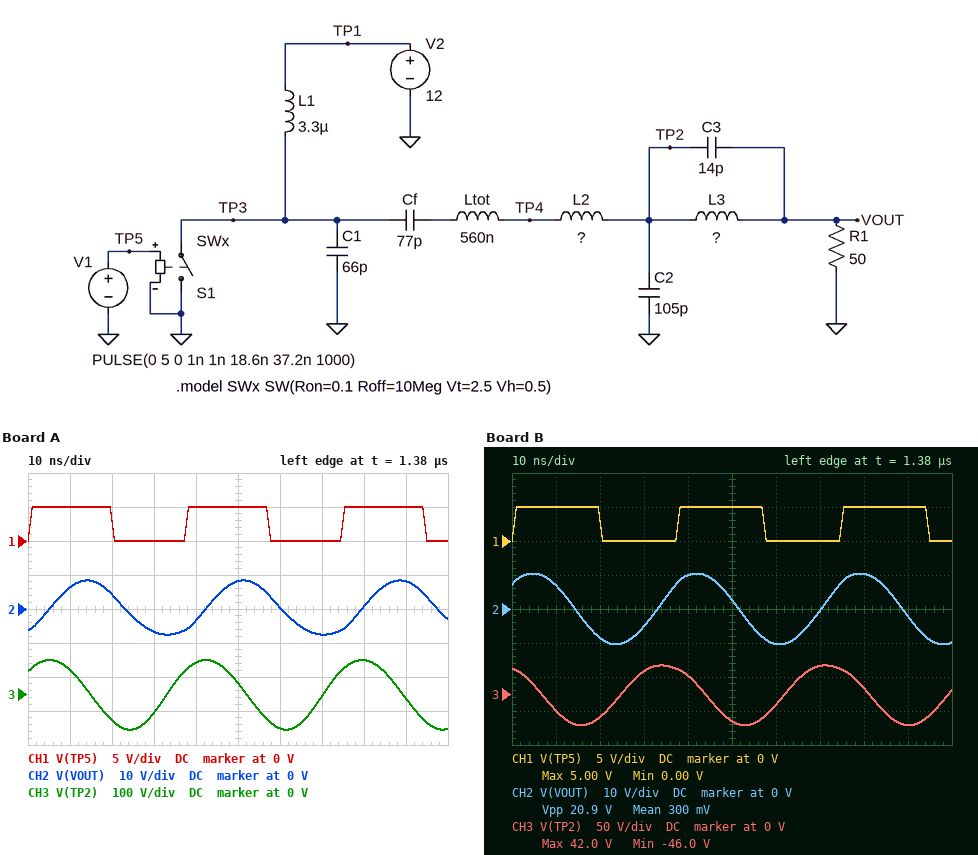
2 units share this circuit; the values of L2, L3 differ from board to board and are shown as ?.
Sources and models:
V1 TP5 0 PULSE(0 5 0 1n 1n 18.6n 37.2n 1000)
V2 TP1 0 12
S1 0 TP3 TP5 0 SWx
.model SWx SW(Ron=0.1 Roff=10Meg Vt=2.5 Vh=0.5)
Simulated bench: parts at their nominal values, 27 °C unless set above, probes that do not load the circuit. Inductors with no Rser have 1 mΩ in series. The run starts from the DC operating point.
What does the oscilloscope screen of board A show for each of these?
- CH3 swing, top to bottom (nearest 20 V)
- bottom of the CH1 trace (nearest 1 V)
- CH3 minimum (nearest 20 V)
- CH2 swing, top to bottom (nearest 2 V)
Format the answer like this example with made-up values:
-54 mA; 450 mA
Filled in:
200 V; 0 V; -100 V; 16 V
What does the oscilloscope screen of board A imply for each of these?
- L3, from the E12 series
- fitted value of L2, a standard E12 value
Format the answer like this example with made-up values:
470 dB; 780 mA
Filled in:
1.5 µH; 390 nH
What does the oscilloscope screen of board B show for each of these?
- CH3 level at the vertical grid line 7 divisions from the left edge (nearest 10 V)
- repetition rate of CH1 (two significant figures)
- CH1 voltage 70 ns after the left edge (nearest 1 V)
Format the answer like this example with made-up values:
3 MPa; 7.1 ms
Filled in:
40 V; 27 MHz; 0 V
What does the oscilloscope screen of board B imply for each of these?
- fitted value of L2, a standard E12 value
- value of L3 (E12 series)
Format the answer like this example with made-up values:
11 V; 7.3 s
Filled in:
150 nH; 820 nH
